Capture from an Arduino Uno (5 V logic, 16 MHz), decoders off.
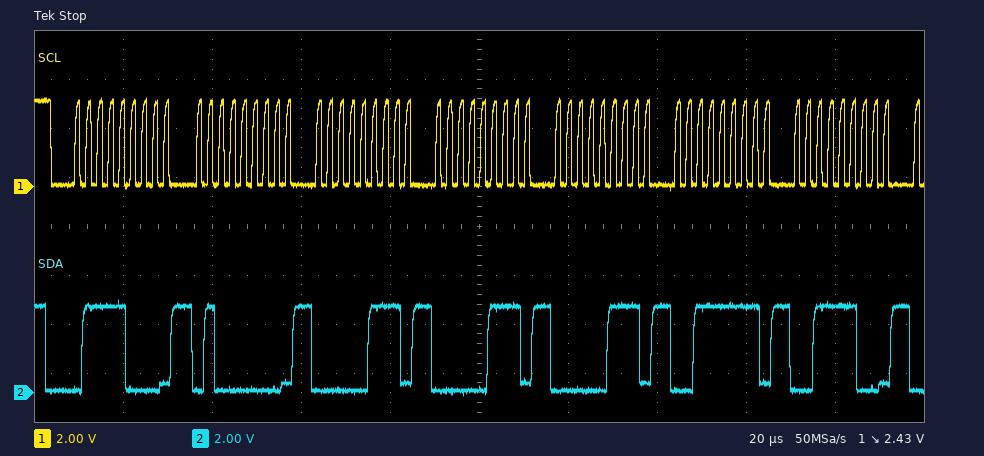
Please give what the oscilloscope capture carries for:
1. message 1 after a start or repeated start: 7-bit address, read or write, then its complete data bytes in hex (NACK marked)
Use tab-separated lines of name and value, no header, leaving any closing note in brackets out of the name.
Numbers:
message 1 after a start or repeated start: 7-bit address, read or write, then its complete data bytes in hex	0x3C write: 40 07 07 07 3F 3C
